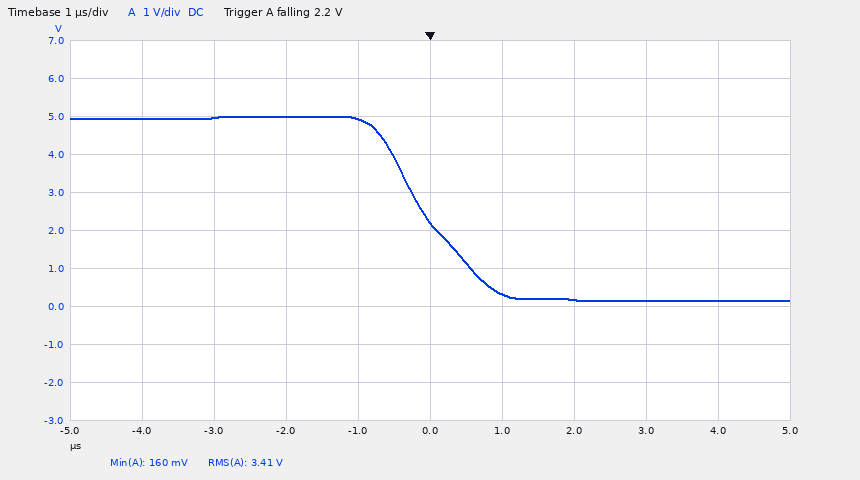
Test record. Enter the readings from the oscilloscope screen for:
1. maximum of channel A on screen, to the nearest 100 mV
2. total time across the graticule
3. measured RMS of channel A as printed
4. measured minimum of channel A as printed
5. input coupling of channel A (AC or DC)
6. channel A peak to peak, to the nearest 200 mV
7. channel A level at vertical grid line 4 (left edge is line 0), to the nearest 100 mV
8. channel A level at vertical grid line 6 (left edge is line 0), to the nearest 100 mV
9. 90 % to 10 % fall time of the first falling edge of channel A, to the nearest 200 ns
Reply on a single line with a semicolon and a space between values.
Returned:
5.0 V; 10 µs; 3.41 V; 160 mV; DC; 4.8 V; 4.9 V; 300 mV; 1.4 µs
